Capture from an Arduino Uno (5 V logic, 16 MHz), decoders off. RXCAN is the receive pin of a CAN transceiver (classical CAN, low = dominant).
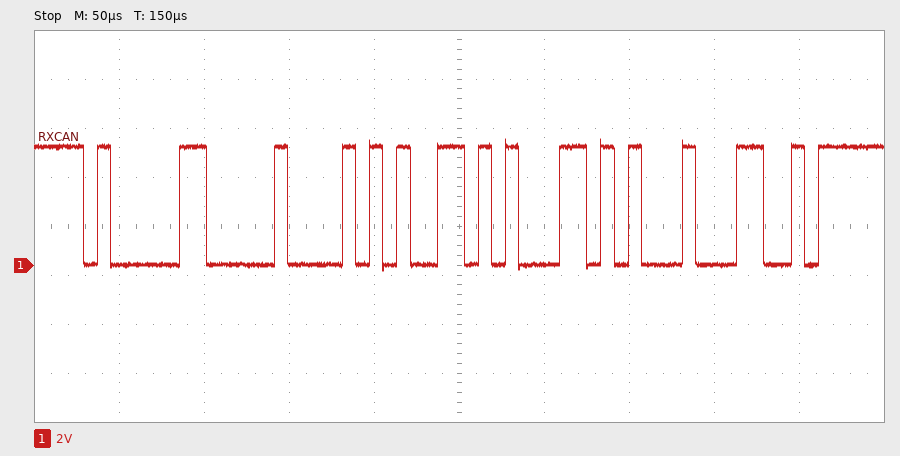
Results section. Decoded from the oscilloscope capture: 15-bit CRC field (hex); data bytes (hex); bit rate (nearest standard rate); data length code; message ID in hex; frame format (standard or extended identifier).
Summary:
0x288C
A6 A3
125 kbit/s
2
0x410
standard
